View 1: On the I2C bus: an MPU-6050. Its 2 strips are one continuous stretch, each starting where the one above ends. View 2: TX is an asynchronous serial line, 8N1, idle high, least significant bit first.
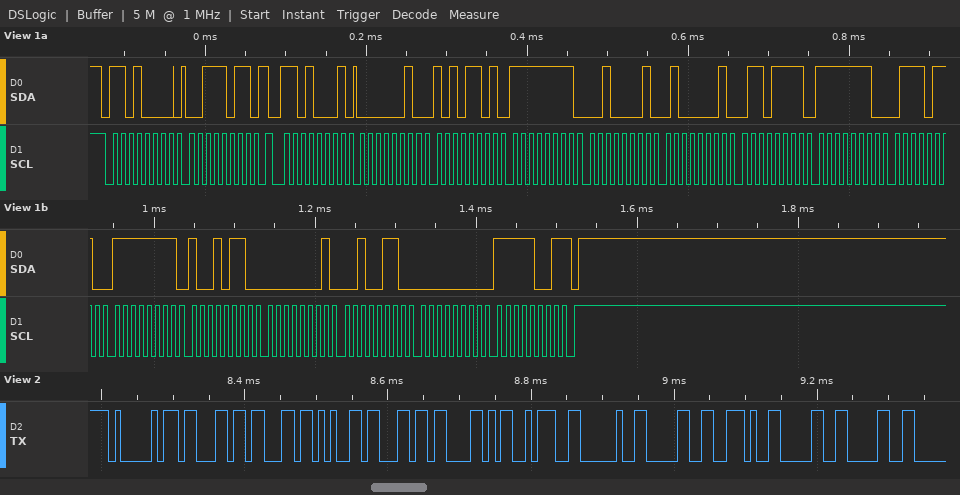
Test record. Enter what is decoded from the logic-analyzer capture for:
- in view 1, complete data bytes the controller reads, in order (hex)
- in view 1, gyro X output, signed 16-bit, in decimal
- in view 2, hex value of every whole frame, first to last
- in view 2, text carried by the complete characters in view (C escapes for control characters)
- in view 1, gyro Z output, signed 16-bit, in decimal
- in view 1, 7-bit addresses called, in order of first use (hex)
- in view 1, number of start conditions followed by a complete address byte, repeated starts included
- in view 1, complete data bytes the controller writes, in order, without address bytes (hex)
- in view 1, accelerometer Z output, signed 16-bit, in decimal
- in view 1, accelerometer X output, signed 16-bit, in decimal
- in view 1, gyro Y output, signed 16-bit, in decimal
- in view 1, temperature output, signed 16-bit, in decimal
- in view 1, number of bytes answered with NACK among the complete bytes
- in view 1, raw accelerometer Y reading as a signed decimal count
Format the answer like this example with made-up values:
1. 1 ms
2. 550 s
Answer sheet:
1. 02 AD FF 21 41 6F FE 76 FF 96 01 26 00 F9
2. -106
3. 41 63 63 65 6C 58 3A 20 30 2E 30 30
4. "AccelX: 0.00"
5. 249
6. 0x68
7. 2
8. 3B
9. 16751
10. 685
11. 294
12. -394
13. 1
14. -223
